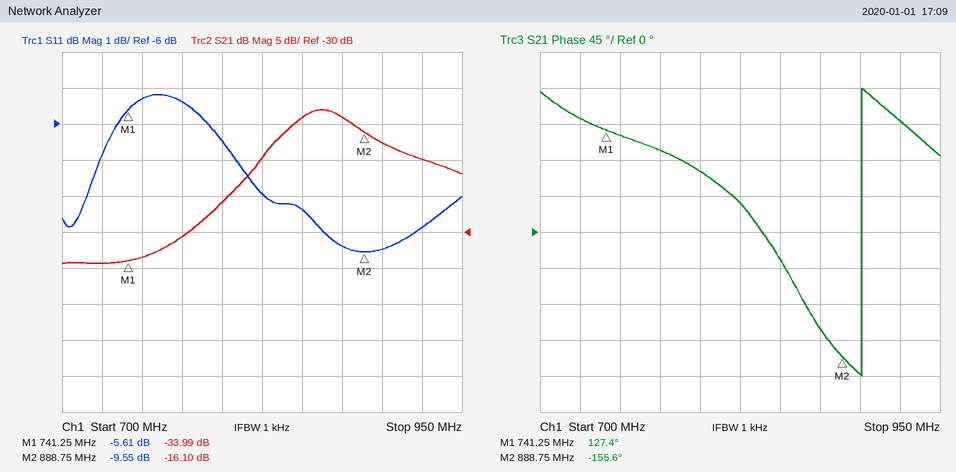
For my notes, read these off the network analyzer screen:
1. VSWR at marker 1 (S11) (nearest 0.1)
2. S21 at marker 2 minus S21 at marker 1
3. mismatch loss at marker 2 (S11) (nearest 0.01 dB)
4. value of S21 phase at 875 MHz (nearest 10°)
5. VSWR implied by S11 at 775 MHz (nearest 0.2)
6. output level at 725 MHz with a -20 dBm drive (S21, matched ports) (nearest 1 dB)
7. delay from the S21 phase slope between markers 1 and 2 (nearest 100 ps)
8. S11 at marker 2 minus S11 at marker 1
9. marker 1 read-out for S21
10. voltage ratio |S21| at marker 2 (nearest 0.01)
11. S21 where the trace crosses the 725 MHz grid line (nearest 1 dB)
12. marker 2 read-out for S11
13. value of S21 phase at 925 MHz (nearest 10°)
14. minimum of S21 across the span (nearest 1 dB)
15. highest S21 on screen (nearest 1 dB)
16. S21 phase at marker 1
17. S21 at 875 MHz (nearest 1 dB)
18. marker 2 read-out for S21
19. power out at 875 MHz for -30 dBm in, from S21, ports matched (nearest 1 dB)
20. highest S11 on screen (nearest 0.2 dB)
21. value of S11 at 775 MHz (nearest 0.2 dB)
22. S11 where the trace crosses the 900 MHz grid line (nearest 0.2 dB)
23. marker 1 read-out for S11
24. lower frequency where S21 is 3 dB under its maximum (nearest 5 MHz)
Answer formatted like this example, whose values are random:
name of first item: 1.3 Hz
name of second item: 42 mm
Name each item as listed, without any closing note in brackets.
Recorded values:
VSWR at marker 1 (S11): 3.2
S21 at marker 2 minus S21 at marker 1: 17.89 dB
mismatch loss at marker 2 (S11): 0.51 dB
value of S21 phase at 875 MHz: -120°
VSWR implied by S11 at 775 MHz: 3.4
output level at 725 MHz with a -20 dBm drive (S21, matched ports): -54 dBm
delay from the S21 phase slope between markers 1 and 2: 5.3 ns
S11 at marker 2 minus S11 at marker 1: -3.94 dB
marker 1 read-out for S21: -33.99 dB
voltage ratio |S21| at marker 2: 0.16
S21 where the trace crosses the 725 MHz grid line: -34 dB
marker 2 read-out for S11: -9.55 dB
value of S21 phase at 925 MHz: 140°
minimum of S21 across the span: -34 dB
highest S21 on screen: -13 dB
S21 phase at marker 1: 127.4°
S21 at 875 MHz: -14 dB
marker 2 read-out for S21: -16.10 dB
power out at 875 MHz for -30 dBm in, from S21, ports matched: -44 dBm
highest S11 on screen: -5.2 dB
value of S11 at 775 MHz: -5.4 dB
S11 where the trace crosses the 900 MHz grid line: -9.4 dB
marker 1 read-out for S11: -5.61 dB
lower frequency where S21 is 3 dB under its maximum: 840 MHz
